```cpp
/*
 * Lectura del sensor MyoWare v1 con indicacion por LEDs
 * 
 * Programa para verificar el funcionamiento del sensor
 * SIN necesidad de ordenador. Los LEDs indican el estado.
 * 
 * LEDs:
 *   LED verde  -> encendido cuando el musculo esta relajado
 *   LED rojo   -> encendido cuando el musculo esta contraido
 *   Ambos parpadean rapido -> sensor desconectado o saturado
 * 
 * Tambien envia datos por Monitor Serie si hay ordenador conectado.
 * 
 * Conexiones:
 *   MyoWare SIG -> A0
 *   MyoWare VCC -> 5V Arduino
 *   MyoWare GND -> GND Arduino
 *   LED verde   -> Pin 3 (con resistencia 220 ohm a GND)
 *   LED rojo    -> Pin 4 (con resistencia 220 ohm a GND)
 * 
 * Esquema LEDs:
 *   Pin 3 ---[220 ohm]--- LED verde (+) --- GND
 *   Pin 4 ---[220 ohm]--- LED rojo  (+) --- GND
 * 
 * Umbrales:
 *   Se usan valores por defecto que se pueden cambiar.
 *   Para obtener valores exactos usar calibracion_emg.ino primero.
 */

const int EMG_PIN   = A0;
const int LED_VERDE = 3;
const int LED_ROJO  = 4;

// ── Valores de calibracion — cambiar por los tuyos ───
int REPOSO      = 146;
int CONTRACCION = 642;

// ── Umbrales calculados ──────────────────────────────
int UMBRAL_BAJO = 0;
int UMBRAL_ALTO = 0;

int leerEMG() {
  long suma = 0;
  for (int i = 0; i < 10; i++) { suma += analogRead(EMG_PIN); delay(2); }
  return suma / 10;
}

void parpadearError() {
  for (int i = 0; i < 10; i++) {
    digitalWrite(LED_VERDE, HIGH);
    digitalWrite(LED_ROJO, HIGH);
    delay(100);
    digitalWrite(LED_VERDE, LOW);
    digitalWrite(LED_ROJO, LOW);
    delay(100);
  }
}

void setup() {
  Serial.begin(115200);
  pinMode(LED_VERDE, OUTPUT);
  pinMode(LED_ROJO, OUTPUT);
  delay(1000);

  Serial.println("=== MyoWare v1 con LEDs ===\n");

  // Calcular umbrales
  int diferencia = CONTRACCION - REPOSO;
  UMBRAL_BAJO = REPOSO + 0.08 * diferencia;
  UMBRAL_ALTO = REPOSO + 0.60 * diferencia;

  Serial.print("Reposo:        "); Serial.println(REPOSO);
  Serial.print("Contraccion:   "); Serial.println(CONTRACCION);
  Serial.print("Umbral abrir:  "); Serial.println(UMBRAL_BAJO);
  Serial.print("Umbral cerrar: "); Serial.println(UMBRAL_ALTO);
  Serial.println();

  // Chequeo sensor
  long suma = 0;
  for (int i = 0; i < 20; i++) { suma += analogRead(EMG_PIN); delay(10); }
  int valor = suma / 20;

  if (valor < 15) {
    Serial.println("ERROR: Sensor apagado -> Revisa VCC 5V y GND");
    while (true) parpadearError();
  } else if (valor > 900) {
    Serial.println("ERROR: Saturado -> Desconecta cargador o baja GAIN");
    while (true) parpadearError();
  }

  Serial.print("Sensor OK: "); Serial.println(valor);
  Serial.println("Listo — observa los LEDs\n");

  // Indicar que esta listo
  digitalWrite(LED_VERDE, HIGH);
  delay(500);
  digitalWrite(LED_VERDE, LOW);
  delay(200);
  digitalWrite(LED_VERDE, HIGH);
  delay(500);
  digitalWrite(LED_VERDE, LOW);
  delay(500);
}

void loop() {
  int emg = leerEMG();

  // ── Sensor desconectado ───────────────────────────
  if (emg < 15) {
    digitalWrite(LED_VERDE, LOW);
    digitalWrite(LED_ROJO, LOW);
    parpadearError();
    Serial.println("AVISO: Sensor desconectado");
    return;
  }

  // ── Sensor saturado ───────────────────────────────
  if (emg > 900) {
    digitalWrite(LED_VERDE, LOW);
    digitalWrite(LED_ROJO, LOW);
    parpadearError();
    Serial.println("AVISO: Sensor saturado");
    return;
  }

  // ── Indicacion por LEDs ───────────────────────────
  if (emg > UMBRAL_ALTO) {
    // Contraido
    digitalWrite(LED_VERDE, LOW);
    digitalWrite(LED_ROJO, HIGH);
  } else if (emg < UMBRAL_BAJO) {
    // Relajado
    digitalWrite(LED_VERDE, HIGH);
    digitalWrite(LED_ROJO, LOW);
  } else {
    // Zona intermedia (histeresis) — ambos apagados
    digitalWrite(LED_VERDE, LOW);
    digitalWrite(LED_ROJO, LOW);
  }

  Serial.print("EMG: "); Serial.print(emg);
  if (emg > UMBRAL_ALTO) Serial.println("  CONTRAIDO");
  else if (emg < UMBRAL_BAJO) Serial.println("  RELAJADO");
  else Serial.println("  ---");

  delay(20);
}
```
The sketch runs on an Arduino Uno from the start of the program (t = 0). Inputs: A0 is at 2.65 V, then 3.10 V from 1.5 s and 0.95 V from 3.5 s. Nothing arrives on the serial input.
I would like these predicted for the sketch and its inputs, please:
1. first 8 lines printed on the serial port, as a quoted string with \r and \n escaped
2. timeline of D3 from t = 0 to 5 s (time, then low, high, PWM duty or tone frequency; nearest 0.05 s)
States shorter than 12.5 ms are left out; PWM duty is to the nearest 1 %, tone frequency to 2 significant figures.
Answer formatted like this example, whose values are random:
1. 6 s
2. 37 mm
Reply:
1. "=== MyoWare v1 con LEDs ===\n\r\nReposo:        146\r\nContraccion:   642\r\nUmbral abrir:  185\r\nUmbral cerrar: 443\r\n\r\nSensor OK: 542\r\n"
2. 0 s low; 1.2 s high; 1.7 s low; 1.9 s high; 2.4 s low
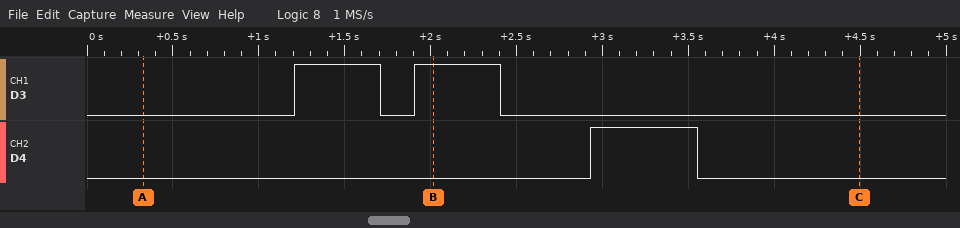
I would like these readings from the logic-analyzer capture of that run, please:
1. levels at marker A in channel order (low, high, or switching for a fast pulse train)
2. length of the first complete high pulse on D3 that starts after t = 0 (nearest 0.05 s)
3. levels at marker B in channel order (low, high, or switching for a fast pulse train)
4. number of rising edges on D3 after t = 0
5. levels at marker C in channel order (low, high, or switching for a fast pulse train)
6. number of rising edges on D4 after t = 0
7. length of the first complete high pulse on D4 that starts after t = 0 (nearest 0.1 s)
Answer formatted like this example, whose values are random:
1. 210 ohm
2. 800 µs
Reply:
1. D3 low, D4 low
2. 0.50 s
3. D3 high, D4 low
4. 2
5. D3 low, D4 low
6. 1
7. 0.6 s
